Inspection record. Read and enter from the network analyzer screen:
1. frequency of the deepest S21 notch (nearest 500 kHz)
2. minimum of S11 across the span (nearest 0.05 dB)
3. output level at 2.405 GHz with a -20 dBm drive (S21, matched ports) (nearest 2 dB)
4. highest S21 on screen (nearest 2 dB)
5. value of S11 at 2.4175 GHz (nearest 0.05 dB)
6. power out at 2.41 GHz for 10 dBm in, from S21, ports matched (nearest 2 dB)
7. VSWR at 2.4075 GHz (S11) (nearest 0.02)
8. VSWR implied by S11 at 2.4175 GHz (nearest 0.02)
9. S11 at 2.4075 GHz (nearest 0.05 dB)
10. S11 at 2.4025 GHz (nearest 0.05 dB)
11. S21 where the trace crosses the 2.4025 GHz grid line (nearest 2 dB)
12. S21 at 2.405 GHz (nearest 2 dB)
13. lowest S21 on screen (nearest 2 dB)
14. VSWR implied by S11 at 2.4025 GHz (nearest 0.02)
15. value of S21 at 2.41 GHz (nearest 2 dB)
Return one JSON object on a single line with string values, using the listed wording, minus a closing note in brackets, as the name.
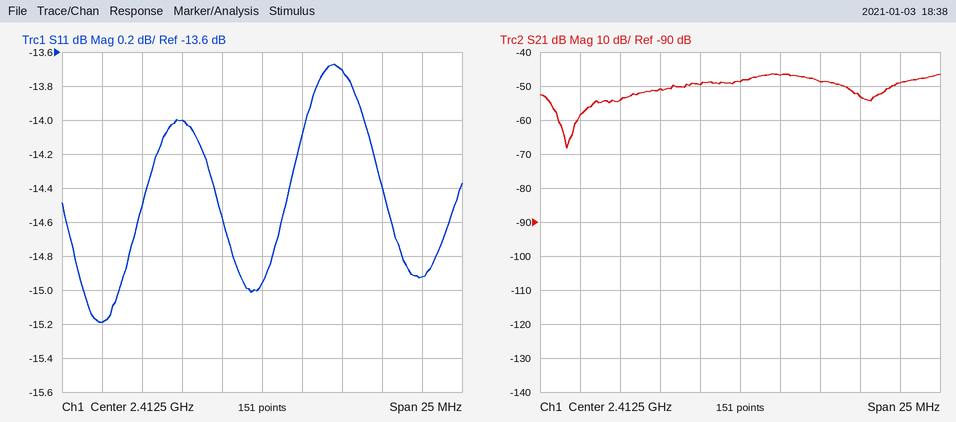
{"frequency of the deepest S21 notch": "2.4015 GHz", "minimum of S11 across the span": "-15.20 dB", "output level at 2.405 GHz with a -20 dBm drive (S21, matched ports)": "-74 dBm", "highest S21 on screen": "-46 dB", "value of S11 at 2.4175 GHz": "-13.70 dB", "power out at 2.41 GHz for 10 dBm in, from S21, ports matched": "-40 dBm", "VSWR at 2.4075 GHz (S11)": "1.50", "VSWR implied by S11 at 2.4175 GHz": "1.52", "S11 at 2.4075 GHz": "-14.00 dB", "S11 at 2.4025 GHz": "-15.20 dB", "S21 where the trace crosses the 2.4025 GHz grid line": "-58 dB", "S21 at 2.405 GHz": "-54 dB", "lowest S21 on screen": "-68 dB", "VSWR implied by S11 at 2.4025 GHz": "1.42", "value of S21 at 2.41 GHz": "-50 dB"}
